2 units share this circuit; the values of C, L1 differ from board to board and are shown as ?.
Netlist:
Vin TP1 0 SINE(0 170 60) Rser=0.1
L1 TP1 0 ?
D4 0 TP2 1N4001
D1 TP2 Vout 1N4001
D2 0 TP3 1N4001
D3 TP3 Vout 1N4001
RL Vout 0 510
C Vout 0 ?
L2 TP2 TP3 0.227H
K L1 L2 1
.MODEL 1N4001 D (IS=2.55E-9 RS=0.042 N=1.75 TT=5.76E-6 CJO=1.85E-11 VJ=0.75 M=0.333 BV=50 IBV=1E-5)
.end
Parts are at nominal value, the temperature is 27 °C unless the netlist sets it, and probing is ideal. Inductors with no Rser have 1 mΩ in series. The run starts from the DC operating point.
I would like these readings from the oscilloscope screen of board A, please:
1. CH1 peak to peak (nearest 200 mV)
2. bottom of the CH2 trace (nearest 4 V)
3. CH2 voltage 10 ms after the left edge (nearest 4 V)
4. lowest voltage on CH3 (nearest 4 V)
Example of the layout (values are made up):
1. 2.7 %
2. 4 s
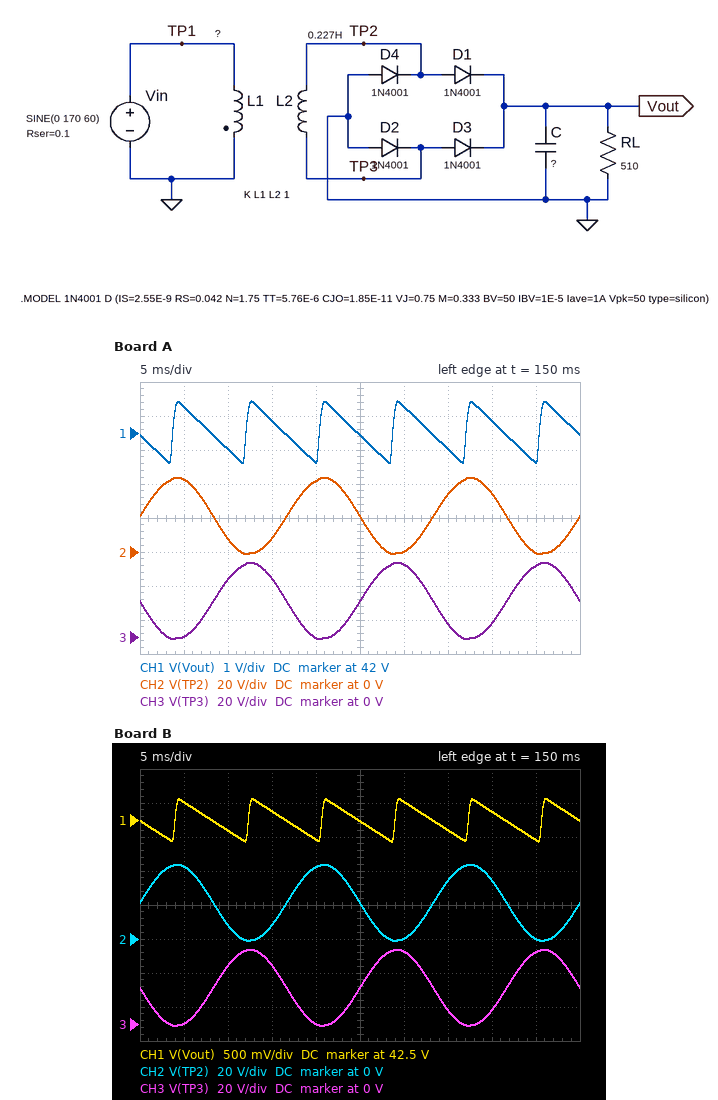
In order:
1. 1.8 V
2. 0 V
3. 8 V
4. 0 V
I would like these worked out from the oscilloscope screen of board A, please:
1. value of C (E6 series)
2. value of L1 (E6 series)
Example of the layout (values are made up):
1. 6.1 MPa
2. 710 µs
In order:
1. 330 µF
2. 3.3 H
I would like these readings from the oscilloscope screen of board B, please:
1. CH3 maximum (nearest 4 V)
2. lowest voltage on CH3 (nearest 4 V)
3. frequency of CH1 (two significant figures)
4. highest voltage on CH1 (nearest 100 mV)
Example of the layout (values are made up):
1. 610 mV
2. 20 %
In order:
1. 44 V
2. 0 V
3. 120 Hz
4. 42.8 V
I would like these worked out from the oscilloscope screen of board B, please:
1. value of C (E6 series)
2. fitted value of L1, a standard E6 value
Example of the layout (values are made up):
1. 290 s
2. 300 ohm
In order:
1. 1 mF
2. 3.3 H
